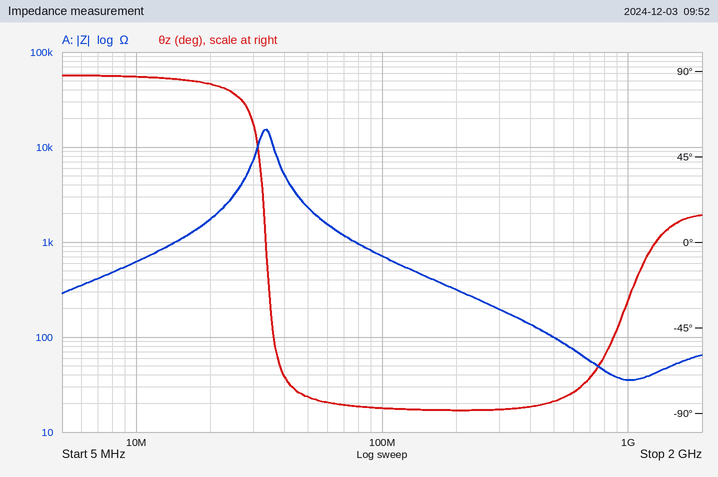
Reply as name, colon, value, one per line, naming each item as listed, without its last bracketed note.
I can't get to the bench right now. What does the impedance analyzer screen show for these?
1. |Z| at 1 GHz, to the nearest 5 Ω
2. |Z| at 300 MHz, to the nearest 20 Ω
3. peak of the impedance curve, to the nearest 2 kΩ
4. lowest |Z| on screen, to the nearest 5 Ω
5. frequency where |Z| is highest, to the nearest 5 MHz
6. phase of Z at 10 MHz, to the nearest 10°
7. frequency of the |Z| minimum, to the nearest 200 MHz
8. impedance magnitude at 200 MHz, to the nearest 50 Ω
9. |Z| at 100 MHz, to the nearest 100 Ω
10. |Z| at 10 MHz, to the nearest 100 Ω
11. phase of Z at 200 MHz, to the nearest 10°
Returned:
|Z| at 1 GHz, to the nearest 5 Ω: 35 Ω
|Z| at 300 MHz, to the nearest 20 Ω: 200 Ω
peak of the impedance curve, to the nearest 2 kΩ: 16 kΩ
lowest |Z| on screen, to the nearest 5 Ω: 35 Ω
frequency where |Z| is highest, to the nearest 5 MHz: 35 MHz
phase of Z at 10 MHz, to the nearest 10°: 90°
frequency of the |Z| minimum, to the nearest 200 MHz: 1.0 GHz
impedance magnitude at 200 MHz, to the nearest 50 Ω: 300 Ω
|Z| at 100 MHz, to the nearest 100 Ω: 700 Ω
|Z| at 10 MHz, to the nearest 100 Ω: 600 Ω
phase of Z at 200 MHz, to the nearest 10°: -90°
